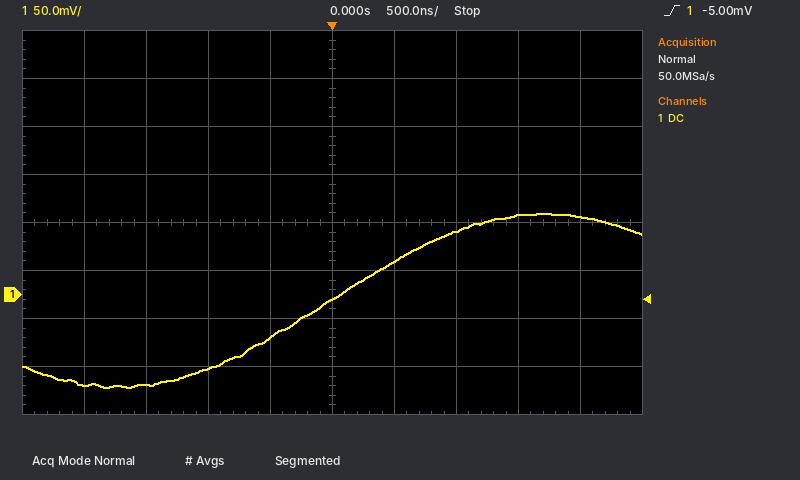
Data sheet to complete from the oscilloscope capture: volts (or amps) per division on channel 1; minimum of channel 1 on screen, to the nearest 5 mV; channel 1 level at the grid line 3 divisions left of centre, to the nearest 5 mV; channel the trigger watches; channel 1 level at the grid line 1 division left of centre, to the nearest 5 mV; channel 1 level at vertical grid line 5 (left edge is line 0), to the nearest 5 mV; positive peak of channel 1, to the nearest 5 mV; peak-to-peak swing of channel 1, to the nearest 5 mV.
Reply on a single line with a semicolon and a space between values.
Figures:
50 mV; -95 mV; -95 mV; channel 1; -45 mV; -5 mV; 85 mV; 180 mV
